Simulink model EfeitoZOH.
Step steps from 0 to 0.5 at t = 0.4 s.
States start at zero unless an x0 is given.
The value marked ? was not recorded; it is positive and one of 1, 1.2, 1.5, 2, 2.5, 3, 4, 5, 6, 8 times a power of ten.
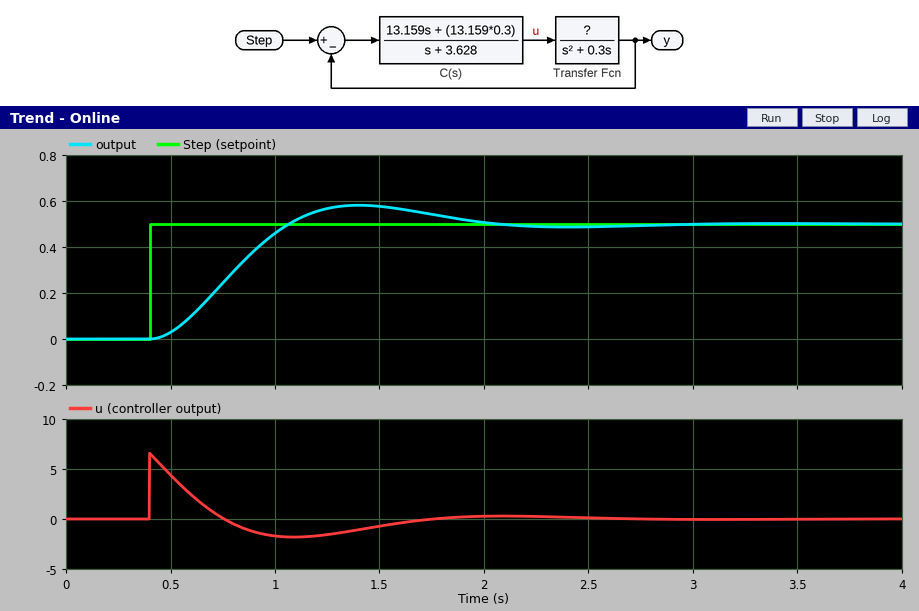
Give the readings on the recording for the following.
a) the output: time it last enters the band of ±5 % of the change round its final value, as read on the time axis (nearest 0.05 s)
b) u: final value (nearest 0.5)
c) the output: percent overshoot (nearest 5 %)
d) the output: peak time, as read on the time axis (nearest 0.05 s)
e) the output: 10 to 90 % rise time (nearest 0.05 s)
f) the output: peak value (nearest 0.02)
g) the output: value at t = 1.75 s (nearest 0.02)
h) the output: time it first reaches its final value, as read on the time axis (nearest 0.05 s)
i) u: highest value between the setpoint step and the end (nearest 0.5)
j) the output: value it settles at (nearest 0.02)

1.85 s
0.0
15 %
1.40 s
0.45 s
0.58
0.54
1.05 s
6.5
0.50
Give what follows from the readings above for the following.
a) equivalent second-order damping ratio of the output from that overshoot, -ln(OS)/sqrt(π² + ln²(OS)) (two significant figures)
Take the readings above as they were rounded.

0.52
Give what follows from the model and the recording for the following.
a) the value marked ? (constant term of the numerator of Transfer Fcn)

1
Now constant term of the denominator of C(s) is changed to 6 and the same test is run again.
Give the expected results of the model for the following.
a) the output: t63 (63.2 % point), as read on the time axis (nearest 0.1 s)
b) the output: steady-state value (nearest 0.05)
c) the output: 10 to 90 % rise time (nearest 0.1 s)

0.9 s
0.50
0.7 s
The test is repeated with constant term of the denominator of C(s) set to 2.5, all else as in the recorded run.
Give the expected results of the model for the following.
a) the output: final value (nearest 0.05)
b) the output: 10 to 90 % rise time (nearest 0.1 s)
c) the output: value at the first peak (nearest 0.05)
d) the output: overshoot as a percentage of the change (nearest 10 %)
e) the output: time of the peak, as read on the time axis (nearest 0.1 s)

0.50
0.4 s
0.65
30 %
1.3 s
